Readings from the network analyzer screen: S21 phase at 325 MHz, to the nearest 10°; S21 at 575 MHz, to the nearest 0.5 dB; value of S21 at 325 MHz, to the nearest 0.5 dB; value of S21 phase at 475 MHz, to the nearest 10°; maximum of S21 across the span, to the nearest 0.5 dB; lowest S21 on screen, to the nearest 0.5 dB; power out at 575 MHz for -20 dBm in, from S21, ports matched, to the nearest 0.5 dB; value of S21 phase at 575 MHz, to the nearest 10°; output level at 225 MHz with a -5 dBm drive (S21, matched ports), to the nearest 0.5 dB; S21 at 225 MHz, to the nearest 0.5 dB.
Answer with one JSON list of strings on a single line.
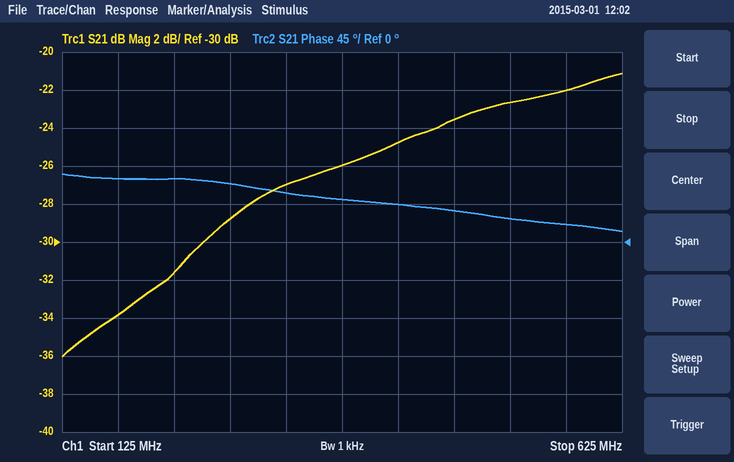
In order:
["60°", "-22.0 dB", "-27.0 dB", "40°", "-21.0 dB", "-36.0 dB", "-42.0 dBm", "20°", "-36.5 dBm", "-31.5 dB"]
